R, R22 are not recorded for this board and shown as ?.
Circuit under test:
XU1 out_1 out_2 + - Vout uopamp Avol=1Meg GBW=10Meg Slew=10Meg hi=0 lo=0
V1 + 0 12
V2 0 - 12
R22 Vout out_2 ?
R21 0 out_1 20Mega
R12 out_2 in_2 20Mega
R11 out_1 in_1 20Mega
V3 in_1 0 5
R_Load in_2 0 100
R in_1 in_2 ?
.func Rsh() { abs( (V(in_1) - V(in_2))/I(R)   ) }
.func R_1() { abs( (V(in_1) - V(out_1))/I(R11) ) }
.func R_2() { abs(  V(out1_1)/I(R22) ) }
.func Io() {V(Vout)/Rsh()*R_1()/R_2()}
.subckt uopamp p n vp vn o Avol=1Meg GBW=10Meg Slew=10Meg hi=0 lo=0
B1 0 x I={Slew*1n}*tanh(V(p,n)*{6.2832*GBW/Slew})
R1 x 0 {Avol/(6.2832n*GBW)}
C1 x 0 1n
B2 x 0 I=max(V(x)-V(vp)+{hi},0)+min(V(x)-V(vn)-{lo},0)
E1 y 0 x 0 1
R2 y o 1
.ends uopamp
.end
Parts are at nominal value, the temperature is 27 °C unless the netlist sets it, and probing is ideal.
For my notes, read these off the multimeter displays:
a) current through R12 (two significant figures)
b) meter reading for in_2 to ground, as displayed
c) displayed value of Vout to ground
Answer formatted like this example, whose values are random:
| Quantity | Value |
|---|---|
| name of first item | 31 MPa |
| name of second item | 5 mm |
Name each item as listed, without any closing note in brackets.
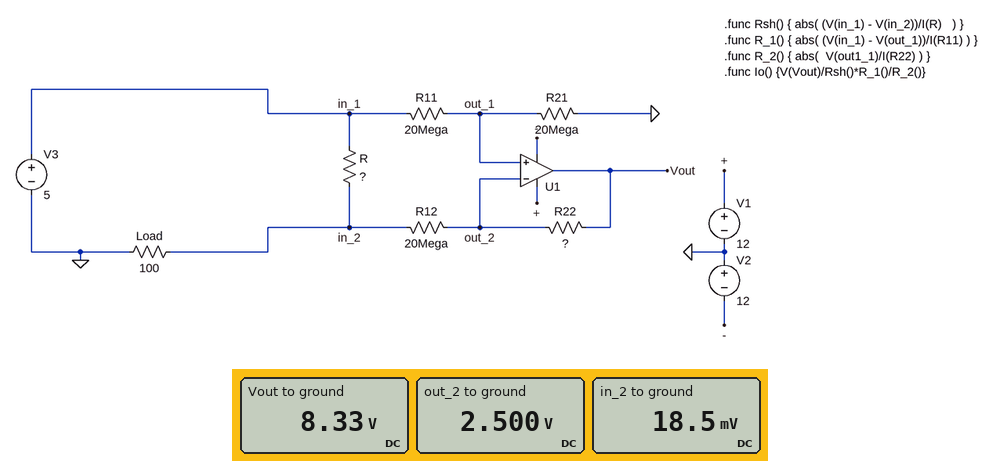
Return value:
| Quantity | Value |
|---|---|
| current through R12 | 120 nA |
| meter reading for in_2 to ground, as displayed | 18.5 mV |
| displayed value of Vout to ground | 8.33 V |
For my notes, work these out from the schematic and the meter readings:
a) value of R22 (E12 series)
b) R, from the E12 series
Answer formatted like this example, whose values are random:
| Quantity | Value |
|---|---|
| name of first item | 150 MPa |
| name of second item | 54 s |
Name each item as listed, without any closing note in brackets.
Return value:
| Quantity | Value |
|---|---|
| value of R22 | 47 MΩ |
| R, from the E12 series | 27 kΩ |
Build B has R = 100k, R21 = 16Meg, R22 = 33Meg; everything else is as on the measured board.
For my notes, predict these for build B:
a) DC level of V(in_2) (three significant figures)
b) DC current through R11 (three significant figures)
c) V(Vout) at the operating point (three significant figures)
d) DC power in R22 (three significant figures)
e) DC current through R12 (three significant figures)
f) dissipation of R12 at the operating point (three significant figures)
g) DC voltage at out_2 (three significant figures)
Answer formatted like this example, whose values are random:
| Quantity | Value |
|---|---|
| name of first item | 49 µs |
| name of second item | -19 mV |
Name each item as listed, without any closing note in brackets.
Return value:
| Quantity | Value |
|---|---|
| DC level of V(in_2) | 5.01 mV |
| DC current through R11 | 139 nA |
| V(Vout) at the operating point | 5.88 V |
| DC power in R22 | 406 nW |
| DC current through R12 | 111 nA |
| dissipation of R12 at the operating point | 246 nW |
| DC voltage at out_2 | 2.22 V |
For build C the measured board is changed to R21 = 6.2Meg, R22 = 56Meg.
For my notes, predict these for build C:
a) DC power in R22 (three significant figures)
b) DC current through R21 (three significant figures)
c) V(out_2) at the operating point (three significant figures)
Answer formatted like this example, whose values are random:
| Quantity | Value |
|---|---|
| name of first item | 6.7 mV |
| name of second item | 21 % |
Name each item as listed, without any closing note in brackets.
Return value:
| Quantity | Value |
|---|---|
| DC power in R22 | 190 nW |
| DC current through R21 | 191 nA |
| V(out_2) at the operating point | 1.18 V |
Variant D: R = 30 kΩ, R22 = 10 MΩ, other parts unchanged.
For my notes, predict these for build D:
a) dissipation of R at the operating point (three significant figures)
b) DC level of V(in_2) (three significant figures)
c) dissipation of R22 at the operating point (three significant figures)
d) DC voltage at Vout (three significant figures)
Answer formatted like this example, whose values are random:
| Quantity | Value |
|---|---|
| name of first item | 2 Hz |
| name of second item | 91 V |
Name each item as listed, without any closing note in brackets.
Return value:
| Quantity | Value |
|---|---|
| dissipation of R at the operating point | 828 µW |
| DC level of V(in_2) | 16.6 mV |
| dissipation of R22 at the operating point | 154 nW |
| DC voltage at Vout | 3.74 V |
